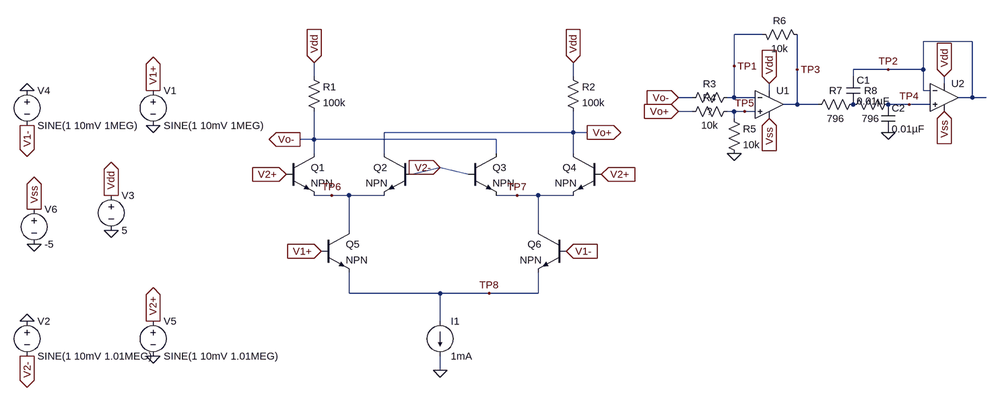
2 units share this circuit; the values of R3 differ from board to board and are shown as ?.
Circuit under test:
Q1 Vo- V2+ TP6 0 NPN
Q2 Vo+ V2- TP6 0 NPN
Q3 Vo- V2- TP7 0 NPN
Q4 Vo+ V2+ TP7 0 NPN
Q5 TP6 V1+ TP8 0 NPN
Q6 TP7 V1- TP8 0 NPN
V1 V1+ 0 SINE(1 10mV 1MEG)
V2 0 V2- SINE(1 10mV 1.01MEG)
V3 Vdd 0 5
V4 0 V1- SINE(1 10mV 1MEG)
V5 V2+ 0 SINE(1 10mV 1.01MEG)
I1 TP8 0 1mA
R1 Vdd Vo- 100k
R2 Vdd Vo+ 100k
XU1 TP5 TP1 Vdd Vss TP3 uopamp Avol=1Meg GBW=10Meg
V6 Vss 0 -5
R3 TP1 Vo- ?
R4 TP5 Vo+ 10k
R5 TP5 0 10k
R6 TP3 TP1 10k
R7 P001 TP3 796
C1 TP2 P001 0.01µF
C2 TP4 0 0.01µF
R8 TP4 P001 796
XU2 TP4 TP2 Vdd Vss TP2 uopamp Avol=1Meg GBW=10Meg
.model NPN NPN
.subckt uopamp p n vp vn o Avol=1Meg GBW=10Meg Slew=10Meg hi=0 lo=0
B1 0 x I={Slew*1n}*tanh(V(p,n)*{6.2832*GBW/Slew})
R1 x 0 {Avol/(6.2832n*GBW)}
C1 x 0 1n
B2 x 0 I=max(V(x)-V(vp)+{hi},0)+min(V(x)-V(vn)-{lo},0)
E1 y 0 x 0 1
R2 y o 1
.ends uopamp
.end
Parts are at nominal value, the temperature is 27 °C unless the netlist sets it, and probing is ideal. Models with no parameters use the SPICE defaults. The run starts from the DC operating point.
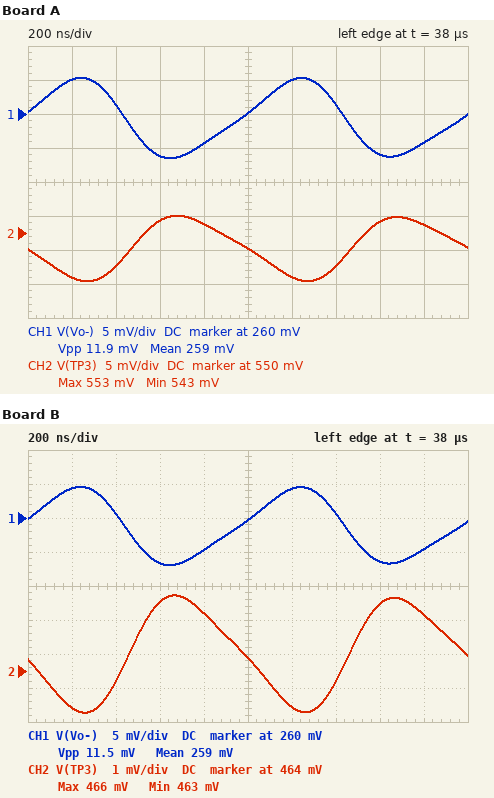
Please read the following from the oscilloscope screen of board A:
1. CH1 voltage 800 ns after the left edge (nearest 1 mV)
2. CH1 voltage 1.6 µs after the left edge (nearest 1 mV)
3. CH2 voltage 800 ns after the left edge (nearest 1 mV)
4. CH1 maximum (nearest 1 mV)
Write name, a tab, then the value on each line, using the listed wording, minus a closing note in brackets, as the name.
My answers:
CH1 voltage 800 ns after the left edge	256 mV
CH1 voltage 1.6 µs after the left edge	254 mV
CH2 voltage 800 ns after the left edge	551 mV
CH1 maximum	265 mV
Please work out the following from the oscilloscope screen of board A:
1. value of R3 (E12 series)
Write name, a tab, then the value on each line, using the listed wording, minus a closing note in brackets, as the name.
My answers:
value of R3	12 kΩ
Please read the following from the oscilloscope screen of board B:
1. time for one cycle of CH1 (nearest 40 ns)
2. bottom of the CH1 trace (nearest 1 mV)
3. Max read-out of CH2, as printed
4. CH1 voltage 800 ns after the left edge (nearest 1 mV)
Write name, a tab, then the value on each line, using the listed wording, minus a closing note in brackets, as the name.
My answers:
time for one cycle of CH1	1.00 µs
bottom of the CH1 trace	253 mV
Max read-out of CH2, as printed	466 mV
CH1 voltage 800 ns after the left edge	255 mV
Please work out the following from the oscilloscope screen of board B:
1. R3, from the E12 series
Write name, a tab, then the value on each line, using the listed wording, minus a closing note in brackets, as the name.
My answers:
R3, from the E12 series	33 kΩ
